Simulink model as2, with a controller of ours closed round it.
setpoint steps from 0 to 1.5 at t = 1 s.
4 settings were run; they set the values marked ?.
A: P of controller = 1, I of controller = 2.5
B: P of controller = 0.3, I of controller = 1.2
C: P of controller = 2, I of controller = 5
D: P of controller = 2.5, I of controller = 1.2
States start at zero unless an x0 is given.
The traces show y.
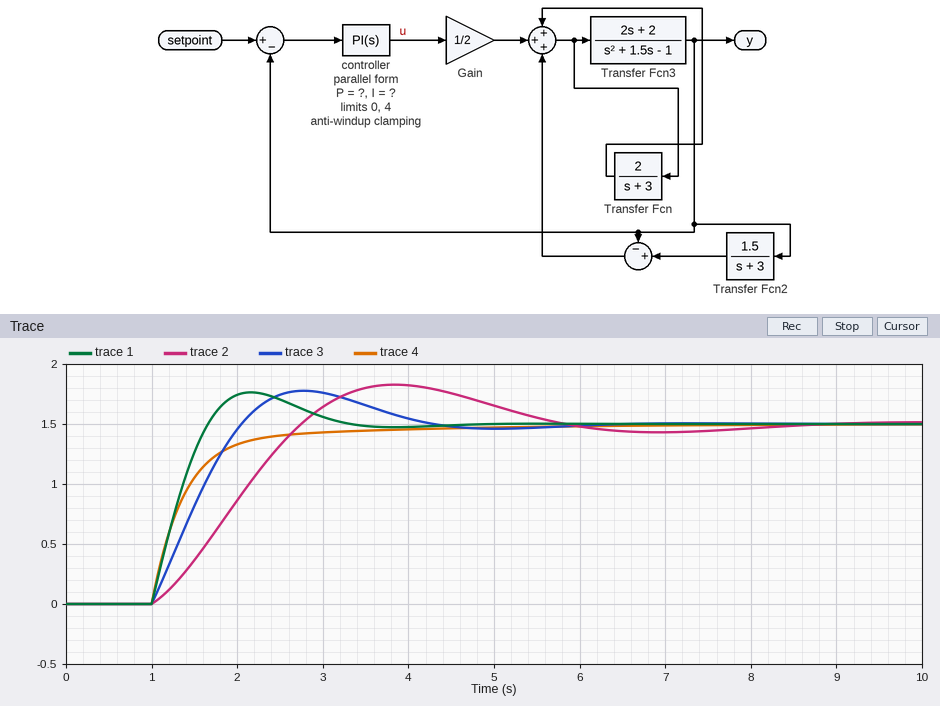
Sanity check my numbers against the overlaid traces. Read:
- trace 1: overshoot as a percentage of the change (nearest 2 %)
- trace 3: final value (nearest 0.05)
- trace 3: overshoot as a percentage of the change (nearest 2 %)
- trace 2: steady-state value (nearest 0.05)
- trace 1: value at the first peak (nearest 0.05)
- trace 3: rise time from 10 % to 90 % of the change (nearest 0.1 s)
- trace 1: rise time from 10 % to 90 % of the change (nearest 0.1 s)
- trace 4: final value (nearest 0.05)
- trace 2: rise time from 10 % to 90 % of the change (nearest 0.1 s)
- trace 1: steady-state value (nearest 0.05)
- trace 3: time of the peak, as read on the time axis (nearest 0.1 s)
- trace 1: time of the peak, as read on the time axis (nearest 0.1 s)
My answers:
18 %
1.50
18 %
1.50
1.75
0.8 s
0.5 s
1.50
1.3 s
1.50
2.8 s
2.2 s
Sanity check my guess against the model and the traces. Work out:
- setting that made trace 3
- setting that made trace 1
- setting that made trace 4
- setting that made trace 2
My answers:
A
C
D
B
